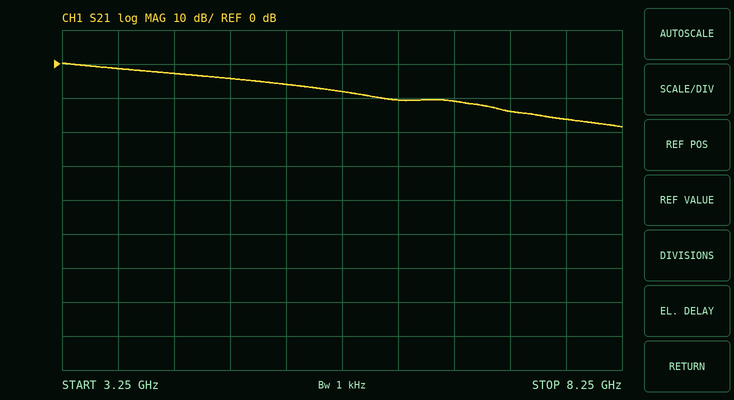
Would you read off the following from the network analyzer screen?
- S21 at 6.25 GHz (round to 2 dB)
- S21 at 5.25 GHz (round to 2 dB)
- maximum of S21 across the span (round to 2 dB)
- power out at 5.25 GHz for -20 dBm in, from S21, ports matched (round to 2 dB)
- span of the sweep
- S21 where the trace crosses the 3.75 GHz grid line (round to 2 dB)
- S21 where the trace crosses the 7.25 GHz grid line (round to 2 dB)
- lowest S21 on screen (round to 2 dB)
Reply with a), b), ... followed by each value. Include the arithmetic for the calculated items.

a) -10 dB
b) -6 dB
c) 0 dB
d) -20 dBm + (-6 dB) = -26 dBm
e) 5 GHz
f) -2 dB
g) -14 dB
h) -18 dB
